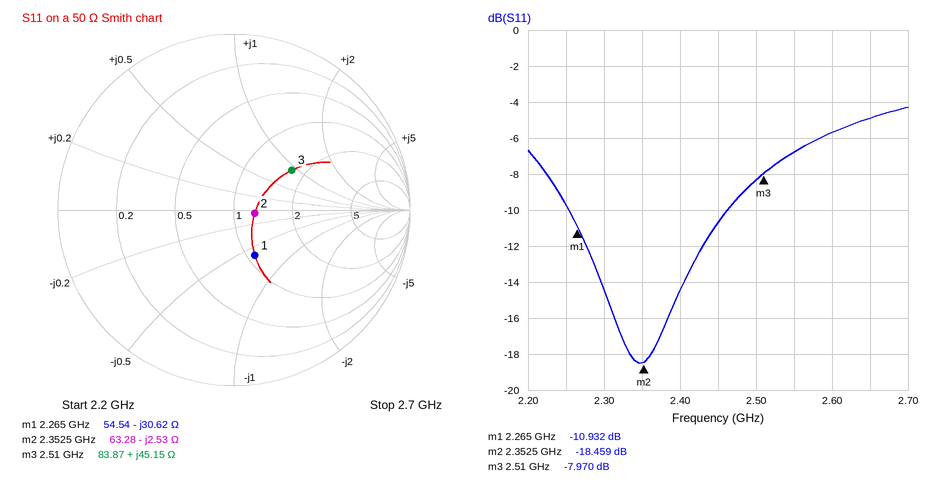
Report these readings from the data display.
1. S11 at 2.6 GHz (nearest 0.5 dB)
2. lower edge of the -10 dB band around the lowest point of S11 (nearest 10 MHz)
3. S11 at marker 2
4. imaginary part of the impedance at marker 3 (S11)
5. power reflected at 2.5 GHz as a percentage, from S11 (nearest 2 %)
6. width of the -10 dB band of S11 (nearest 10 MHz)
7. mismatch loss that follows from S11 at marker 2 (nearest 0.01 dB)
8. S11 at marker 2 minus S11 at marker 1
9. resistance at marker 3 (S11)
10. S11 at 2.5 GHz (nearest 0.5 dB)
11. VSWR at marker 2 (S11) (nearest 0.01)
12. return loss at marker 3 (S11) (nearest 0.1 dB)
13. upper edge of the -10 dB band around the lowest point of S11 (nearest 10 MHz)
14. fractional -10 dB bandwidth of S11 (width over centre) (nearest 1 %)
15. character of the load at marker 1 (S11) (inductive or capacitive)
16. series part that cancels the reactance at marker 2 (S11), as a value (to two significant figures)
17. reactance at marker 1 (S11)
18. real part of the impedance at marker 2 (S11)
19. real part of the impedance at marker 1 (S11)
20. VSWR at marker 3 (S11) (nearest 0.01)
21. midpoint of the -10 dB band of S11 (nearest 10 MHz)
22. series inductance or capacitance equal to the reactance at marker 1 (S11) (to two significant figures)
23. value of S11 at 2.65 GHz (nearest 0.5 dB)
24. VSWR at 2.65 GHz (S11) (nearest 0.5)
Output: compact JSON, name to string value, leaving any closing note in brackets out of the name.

{"S11 at 2.6 GHz": "-5.5 dB", "lower edge of the -10 dB band around the lowest point of S11": "2.25 GHz", "S11 at marker 2": "-18.459 dB", "imaginary part of the impedance at marker 3": "+45.15 Ω", "power reflected at 2.5 GHz as a percentage, from S11": "14 %", "width of the -10 dB band of S11": "210 MHz", "mismatch loss that follows from S11 at marker 2": "0.06 dB", "S11 at marker 2 minus S11 at marker 1": "-7.527 dB", "resistance at marker 3": "83.87 Ω", "S11 at 2.5 GHz": "-8.5 dB", "VSWR at marker 2 (S11)": "1.27", "return loss at marker 3 (S11)": "8.0 dB", "upper edge of the -10 dB band around the lowest point of S11": "2.46 GHz", "fractional -10 dB bandwidth of S11 (width over centre)": "9 %", "character of the load at marker 1 (S11)": "capacitive", "series part that cancels the reactance at marker 2 (S11), as a value": "170 pH", "reactance at marker 1": "-30.62 Ω", "real part of the impedance at marker 2": "63.28 Ω", "real part of the impedance at marker 1": "54.54 Ω", "VSWR at marker 3 (S11)": "2.33", "midpoint of the -10 dB band of S11": "2.36 GHz", "series inductance or capacitance equal to the reactance at marker 1 (S11)": "2.3 pF", "value of S11 at 2.65 GHz": "-5.0 dB", "VSWR at 2.65 GHz (S11)": "3.5"}
